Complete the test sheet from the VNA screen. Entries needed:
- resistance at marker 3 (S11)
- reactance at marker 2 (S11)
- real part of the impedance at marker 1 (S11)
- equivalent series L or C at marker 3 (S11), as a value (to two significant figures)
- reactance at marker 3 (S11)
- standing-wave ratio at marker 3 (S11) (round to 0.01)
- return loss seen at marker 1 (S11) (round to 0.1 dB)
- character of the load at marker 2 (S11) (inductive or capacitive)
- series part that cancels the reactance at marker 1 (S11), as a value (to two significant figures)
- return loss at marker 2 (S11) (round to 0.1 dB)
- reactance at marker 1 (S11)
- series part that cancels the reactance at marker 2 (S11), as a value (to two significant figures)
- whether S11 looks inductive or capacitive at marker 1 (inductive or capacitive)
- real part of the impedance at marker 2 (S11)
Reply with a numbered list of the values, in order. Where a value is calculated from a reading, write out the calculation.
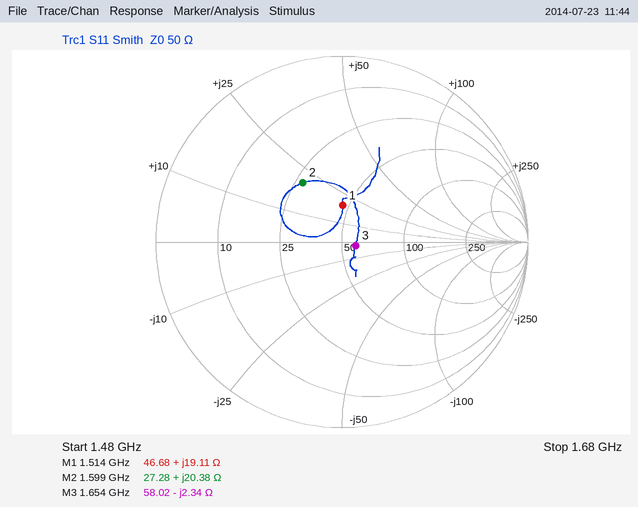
1. 58.02 Ω
2. +20.38 Ω
3. 46.68 Ω
4. C = 1/(2π × 1.654 GHz × 2.34 Ω) ≈ 41 pF
5. -2.34 Ω
6. 1.17
7. 14.1 dB
8. inductive
9. C = 1/(2π × 1.514 GHz × 19.11 Ω) ≈ 5.5 pF
10. 8.4 dB
11. +19.11 Ω
12. C = 1/(2π × 1.599 GHz × 20.38 Ω) ≈ 4.9 pF
13. inductive
14. 27.28 Ω
